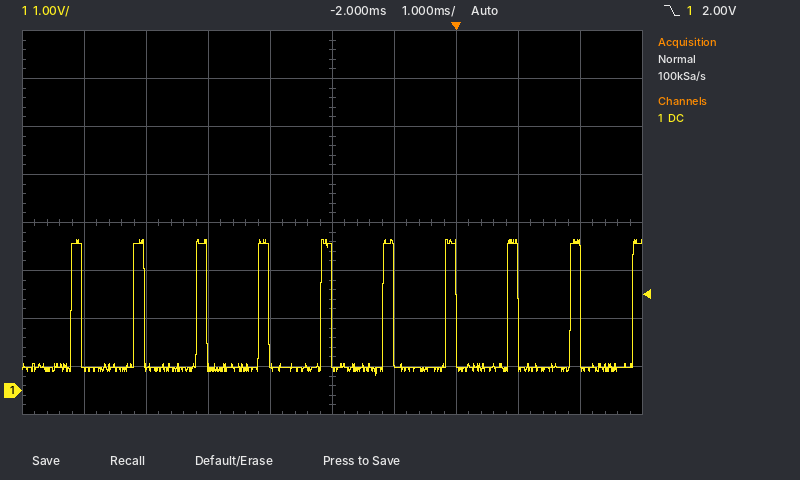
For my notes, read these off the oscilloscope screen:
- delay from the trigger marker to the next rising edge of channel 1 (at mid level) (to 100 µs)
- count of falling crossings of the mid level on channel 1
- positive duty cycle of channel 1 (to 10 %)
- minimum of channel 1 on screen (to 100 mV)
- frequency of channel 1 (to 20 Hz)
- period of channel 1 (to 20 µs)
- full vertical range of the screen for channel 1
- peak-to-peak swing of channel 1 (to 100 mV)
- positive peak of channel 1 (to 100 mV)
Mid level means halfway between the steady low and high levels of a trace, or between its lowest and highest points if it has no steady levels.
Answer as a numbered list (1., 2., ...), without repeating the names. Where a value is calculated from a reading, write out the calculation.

1. 800 µs
2. 9
3. 20 %
4. 300 mV
5. 1 / 1.00 ms ≈ 1.00 kHz
6. 1.00 ms
7. 8 V
8. 3.1 V − (300 mV) = 2.8 V
9. 3.1 V
